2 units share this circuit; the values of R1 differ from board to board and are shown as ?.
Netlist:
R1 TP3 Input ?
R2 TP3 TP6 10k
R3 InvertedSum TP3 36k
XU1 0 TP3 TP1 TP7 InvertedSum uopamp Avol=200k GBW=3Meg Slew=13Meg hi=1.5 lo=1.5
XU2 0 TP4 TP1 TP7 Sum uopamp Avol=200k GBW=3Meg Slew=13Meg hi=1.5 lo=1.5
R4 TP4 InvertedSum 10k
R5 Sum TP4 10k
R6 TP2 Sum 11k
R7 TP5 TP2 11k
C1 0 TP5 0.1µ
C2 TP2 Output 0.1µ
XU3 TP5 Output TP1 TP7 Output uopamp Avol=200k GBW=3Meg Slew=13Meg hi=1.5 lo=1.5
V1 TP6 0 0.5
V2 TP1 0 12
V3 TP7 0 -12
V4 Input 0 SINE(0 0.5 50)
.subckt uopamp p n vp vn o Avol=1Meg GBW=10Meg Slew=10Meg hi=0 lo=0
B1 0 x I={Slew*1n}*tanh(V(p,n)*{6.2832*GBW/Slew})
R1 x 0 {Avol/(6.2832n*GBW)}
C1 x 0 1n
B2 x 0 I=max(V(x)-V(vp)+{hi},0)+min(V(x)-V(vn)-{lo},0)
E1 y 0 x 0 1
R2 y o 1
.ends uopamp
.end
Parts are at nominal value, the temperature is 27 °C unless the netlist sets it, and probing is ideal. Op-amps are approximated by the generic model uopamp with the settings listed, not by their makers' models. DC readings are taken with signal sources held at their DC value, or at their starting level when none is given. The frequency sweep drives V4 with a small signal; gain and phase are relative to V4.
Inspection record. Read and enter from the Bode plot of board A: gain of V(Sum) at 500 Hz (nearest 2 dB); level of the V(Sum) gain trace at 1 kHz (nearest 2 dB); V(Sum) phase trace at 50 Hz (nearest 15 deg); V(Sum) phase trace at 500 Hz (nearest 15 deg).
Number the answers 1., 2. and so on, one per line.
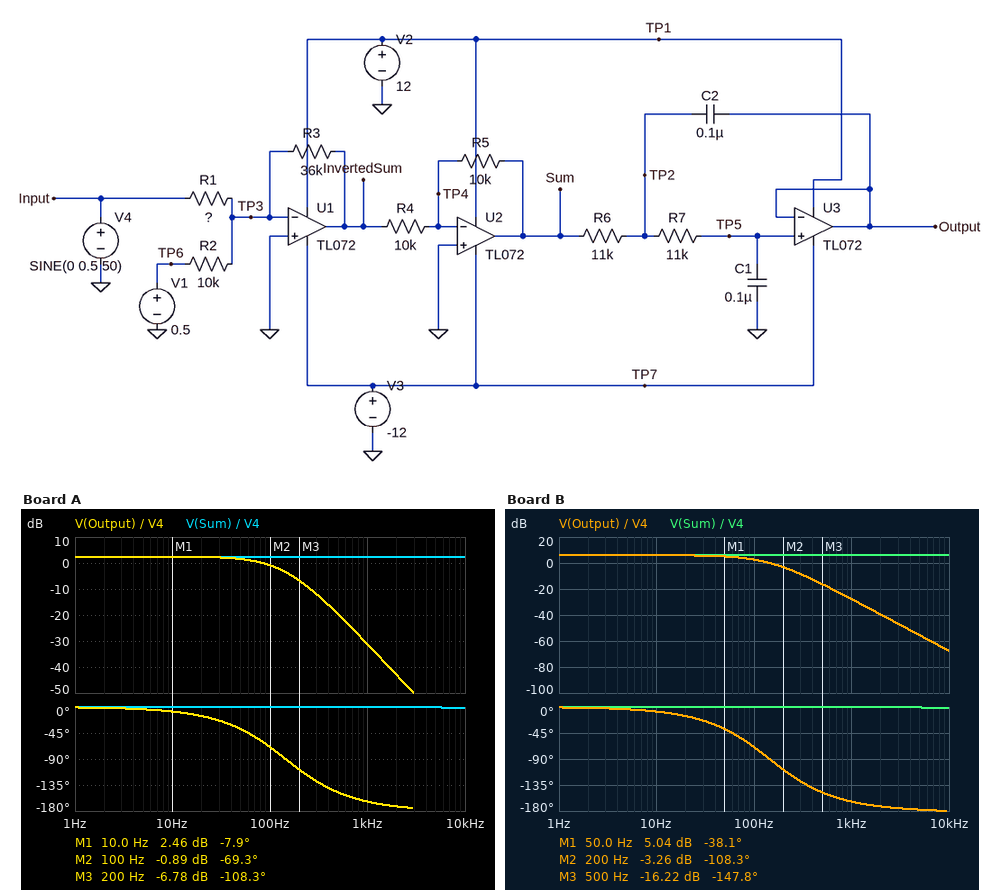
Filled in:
1. 2 dB
2. 2 dB
3. 0 deg
4. 0 deg
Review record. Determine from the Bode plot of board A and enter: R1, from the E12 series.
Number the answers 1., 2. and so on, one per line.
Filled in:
1. 27 kΩ
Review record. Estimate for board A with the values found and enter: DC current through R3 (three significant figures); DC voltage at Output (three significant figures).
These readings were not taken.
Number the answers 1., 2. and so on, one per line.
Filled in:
1. 50.0 µA
2. 1.80 V
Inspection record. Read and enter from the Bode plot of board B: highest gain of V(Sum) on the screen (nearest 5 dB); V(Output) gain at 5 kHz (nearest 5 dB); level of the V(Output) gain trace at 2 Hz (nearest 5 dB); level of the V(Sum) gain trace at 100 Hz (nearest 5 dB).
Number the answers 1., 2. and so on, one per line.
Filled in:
1. 5 dB
2. -55 dB
3. 5 dB
4. 5 dB
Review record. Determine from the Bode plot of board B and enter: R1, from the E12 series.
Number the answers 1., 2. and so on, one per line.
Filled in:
1. 18 kΩ
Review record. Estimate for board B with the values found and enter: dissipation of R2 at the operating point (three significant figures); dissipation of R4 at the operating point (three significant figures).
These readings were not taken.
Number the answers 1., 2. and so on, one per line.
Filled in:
1. 25.0 µW
2. 324 µW
